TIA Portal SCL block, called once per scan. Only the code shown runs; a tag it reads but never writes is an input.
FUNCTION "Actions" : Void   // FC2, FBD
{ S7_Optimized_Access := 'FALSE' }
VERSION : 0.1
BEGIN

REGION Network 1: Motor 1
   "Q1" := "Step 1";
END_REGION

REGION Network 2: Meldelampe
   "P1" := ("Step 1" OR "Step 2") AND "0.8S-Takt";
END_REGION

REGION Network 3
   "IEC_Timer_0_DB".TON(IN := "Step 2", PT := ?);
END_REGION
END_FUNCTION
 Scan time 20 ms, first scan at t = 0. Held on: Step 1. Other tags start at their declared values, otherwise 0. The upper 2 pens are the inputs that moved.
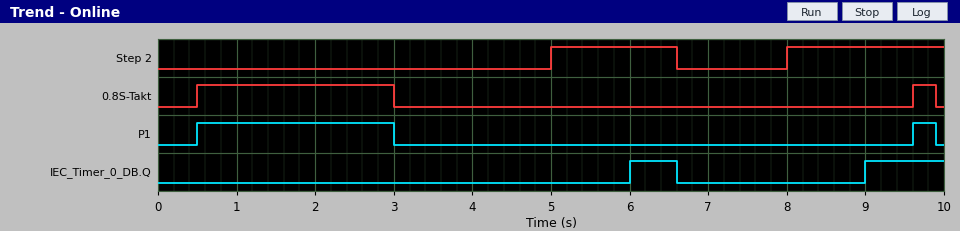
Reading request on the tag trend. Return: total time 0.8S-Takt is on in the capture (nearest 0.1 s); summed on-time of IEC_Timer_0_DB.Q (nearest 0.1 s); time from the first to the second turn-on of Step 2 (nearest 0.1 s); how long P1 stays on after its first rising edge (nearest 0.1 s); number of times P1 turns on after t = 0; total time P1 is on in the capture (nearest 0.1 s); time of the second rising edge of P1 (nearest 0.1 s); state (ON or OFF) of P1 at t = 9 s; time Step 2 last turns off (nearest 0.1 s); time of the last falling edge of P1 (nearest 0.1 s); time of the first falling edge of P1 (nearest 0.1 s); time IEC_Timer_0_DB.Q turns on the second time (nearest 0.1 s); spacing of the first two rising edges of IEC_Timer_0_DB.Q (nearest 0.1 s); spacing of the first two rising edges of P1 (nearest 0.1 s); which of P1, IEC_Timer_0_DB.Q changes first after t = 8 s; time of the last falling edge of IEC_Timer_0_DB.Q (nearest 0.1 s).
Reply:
2.8 s
1.6 s
3.0 s
2.5 s
2
2.8 s
9.6 s
OFF
6.6 s
9.9 s
3.0 s
9.0 s
3.0 s
9.1 s
IEC_Timer_0_DB.Q
6.6 s
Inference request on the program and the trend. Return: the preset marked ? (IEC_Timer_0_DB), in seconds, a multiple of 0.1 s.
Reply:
1.0 s
